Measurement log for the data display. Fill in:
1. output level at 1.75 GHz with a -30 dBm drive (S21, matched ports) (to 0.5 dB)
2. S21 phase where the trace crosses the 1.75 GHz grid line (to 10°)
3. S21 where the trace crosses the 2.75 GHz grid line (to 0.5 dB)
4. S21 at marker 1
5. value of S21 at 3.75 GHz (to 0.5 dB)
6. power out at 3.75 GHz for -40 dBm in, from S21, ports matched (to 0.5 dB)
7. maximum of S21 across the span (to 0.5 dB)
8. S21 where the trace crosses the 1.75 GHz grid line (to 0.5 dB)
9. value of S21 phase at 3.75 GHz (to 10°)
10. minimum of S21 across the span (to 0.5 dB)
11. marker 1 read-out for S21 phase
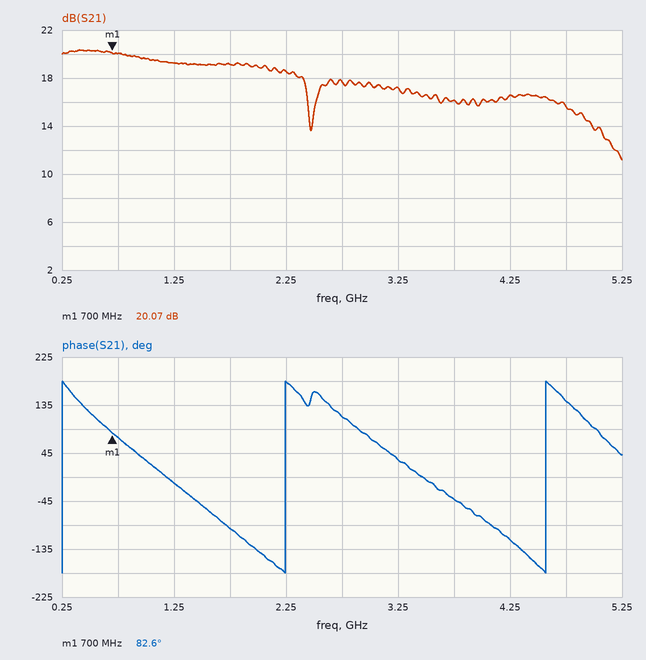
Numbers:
-11.0 dBm
-100°
17.5 dB
20.07 dB
16.0 dB
-24.0 dBm
20.5 dB
19.0 dB
-40°
11.0 dB
82.6°
